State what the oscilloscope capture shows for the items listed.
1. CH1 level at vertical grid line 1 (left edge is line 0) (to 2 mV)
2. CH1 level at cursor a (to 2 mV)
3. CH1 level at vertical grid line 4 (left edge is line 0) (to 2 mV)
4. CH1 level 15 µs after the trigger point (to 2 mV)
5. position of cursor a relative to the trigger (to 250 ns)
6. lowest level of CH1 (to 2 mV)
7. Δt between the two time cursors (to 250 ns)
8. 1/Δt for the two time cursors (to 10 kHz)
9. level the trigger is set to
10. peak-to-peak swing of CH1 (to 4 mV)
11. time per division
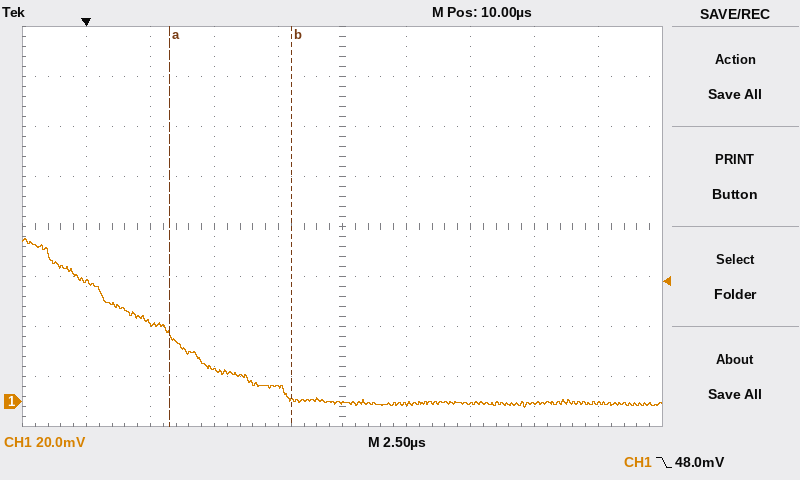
48 mV
26 mV
6 mV
0 mV
+3.25 µs
-2 mV
4.75 µs
210 kHz
48.0 mV
68 mV
2.5 µs
